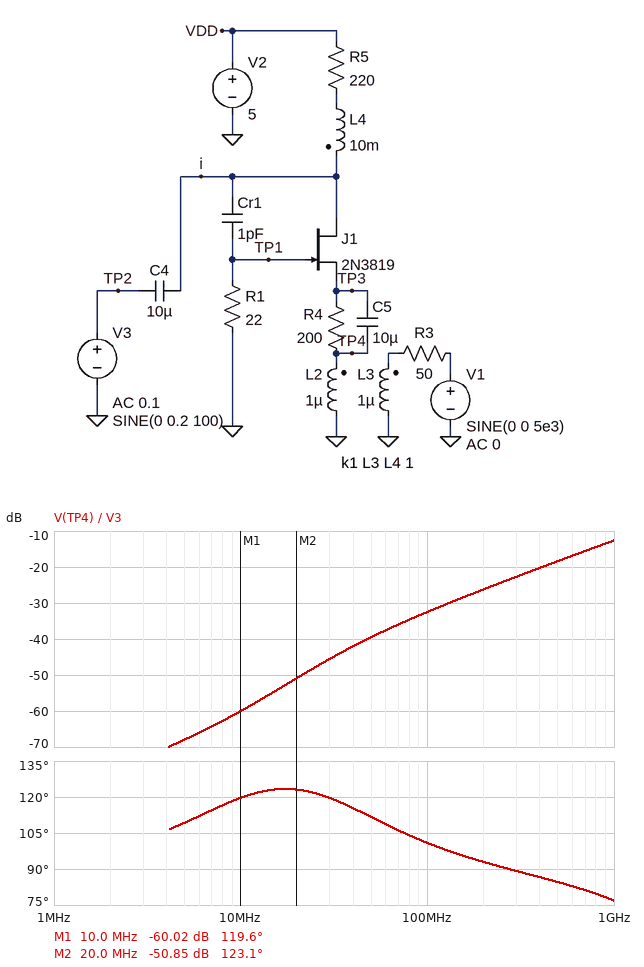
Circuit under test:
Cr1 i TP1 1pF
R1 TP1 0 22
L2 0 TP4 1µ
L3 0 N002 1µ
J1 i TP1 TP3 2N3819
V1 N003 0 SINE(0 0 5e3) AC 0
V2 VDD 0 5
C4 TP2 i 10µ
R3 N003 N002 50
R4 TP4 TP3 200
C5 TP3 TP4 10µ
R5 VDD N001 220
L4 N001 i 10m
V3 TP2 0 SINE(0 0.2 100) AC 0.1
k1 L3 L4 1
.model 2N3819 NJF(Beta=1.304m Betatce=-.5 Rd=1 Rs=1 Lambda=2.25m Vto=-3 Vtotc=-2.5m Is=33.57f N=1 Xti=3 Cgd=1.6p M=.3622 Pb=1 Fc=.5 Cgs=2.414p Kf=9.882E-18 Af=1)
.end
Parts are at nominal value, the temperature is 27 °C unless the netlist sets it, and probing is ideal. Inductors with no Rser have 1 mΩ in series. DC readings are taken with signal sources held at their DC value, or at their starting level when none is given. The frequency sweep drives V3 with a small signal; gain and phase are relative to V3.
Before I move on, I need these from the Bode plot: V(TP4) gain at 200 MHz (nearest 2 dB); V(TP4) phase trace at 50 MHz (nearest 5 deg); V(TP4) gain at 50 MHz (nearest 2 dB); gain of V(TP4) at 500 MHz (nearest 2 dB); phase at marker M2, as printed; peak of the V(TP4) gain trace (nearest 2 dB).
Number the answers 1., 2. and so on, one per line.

1. -26 dB
2. 110 deg
3. -40 dB
4. -18 dB
5. 123.1 deg
6. -12 dB
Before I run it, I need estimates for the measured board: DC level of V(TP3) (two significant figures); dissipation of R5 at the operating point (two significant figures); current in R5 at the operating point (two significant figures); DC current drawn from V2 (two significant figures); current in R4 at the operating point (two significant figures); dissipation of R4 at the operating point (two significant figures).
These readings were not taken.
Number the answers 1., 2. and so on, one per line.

1. 1.0 V
2. 5.7 mW
3. 5.1 mA
4. 5.1 mA
5. 5.1 mA
6. 5.2 mW
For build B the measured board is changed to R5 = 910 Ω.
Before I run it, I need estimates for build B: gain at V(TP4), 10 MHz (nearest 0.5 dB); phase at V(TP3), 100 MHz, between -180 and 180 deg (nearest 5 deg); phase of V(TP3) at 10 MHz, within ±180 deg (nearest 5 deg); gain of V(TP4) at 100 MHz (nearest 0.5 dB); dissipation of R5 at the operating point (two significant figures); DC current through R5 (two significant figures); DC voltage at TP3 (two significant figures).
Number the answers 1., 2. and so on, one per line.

1. -13.0 dB
2. 5 deg
3. 70 deg
4. -4.0 dB
5. 13 mW
6. 3.8 mA
7. 760 mV
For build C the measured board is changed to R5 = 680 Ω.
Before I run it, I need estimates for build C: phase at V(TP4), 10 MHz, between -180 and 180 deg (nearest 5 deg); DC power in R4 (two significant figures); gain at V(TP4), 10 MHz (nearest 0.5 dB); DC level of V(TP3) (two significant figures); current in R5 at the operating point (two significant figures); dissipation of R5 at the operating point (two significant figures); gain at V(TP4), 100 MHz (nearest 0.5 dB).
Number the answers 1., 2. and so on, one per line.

1. 70 deg
2. 3.9 mW
3. -16.0 dB
4. 890 mV
5. 4.4 mA
6. 13 mW
7. -6.5 dB
